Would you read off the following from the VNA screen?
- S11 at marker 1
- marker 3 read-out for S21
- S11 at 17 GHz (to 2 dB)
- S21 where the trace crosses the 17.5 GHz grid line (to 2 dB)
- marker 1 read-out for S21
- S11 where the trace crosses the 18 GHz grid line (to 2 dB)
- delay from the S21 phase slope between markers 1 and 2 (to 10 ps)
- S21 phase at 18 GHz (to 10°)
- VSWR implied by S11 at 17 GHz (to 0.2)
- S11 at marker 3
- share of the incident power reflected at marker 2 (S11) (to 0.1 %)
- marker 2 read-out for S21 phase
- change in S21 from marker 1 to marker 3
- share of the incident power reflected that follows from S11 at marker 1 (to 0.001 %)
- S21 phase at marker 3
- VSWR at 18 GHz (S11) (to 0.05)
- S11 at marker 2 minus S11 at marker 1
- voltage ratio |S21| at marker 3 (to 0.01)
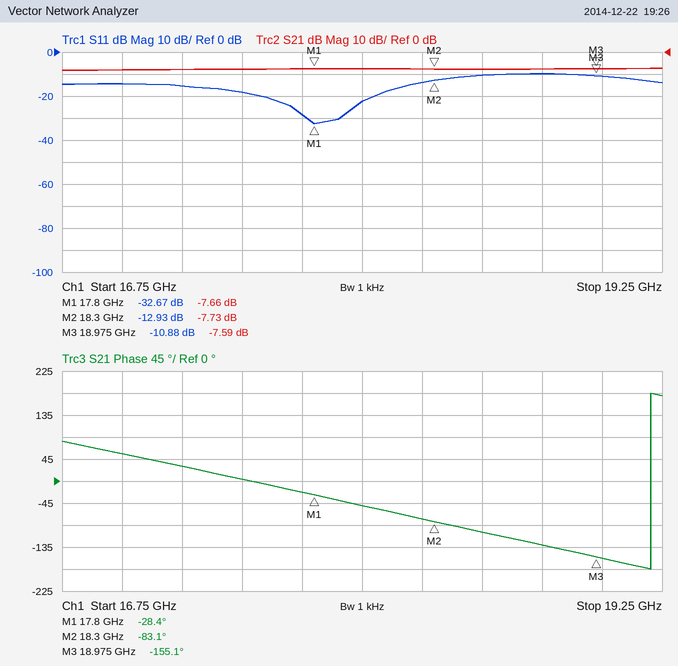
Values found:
-32.67 dB
-7.59 dB
-14 dB
-8 dB
-7.66 dB
-22 dB
300 ps
-50°
1.4
-10.88 dB
5.1 %
-83.1°
0.07 dB
0.054 %
-155.1°
1.15
19.74 dB
0.42
